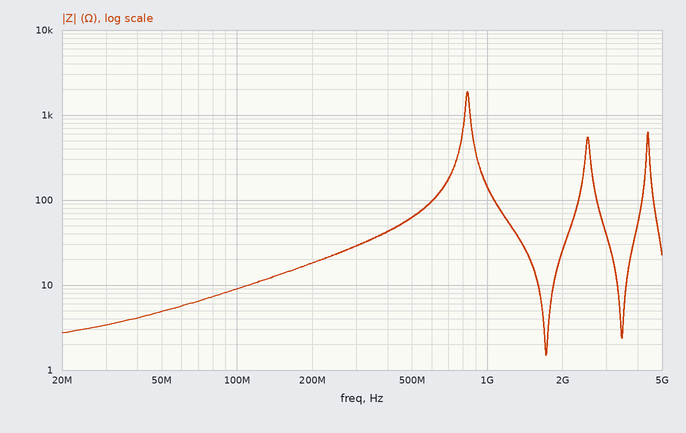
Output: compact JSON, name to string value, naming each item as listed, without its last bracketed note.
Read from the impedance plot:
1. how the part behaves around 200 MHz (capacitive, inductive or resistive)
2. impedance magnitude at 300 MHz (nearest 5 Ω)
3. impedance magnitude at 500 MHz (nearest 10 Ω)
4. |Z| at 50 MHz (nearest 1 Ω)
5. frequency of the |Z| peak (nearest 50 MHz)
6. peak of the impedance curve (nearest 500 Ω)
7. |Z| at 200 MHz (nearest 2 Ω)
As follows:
{"how the part behaves around 200 MHz": "inductive", "impedance magnitude at 300 MHz": "30 Ω", "impedance magnitude at 500 MHz": "60 Ω", "|Z| at 50 MHz": "5 Ω", "frequency of the |Z| peak": "850 MHz", "peak of the impedance curve": "2.0 kΩ", "|Z| at 200 MHz": "18 Ω"}
